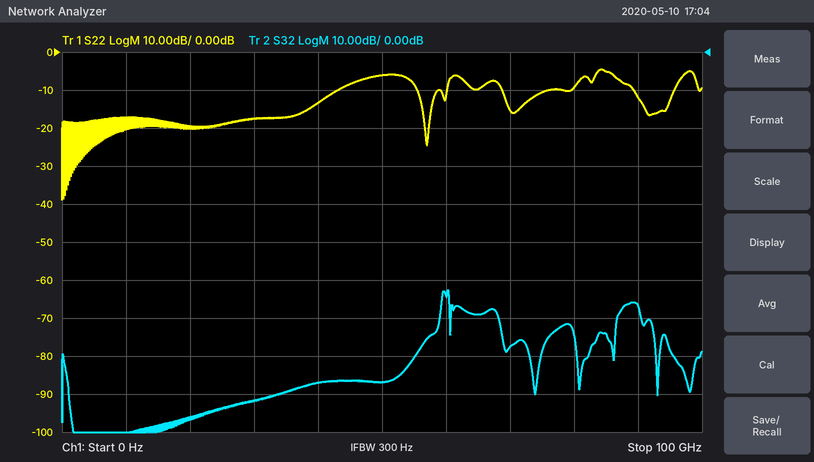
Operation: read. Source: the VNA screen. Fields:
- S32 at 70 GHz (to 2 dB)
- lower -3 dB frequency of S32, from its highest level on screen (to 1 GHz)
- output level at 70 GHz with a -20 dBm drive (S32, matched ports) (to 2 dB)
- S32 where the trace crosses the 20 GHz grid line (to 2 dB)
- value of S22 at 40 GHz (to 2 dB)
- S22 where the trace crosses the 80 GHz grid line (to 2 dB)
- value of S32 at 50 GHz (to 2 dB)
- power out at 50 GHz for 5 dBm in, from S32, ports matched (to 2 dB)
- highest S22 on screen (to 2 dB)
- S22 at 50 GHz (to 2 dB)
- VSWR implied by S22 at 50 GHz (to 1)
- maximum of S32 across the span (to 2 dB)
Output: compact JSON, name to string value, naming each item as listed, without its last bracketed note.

{"S32 at 70 GHz": "-78 dB", "lower -3 dB frequency of S32, from its highest level on screen": "59 GHz", "output level at 70 GHz with a -20 dBm drive (S32, matched ports)": "-98 dBm", "S32 where the trace crosses the 20 GHz grid line": "-96 dB", "value of S22 at 40 GHz": "-14 dB", "S22 where the trace crosses the 80 GHz grid line": "-10 dB", "value of S32 at 50 GHz": "-86 dB", "power out at 50 GHz for 5 dBm in, from S32, ports matched": "-82 dBm", "highest S22 on screen": "-4 dB", "S22 at 50 GHz": "-6 dB", "VSWR implied by S22 at 50 GHz": "3", "maximum of S32 across the span": "-62 dB"}
